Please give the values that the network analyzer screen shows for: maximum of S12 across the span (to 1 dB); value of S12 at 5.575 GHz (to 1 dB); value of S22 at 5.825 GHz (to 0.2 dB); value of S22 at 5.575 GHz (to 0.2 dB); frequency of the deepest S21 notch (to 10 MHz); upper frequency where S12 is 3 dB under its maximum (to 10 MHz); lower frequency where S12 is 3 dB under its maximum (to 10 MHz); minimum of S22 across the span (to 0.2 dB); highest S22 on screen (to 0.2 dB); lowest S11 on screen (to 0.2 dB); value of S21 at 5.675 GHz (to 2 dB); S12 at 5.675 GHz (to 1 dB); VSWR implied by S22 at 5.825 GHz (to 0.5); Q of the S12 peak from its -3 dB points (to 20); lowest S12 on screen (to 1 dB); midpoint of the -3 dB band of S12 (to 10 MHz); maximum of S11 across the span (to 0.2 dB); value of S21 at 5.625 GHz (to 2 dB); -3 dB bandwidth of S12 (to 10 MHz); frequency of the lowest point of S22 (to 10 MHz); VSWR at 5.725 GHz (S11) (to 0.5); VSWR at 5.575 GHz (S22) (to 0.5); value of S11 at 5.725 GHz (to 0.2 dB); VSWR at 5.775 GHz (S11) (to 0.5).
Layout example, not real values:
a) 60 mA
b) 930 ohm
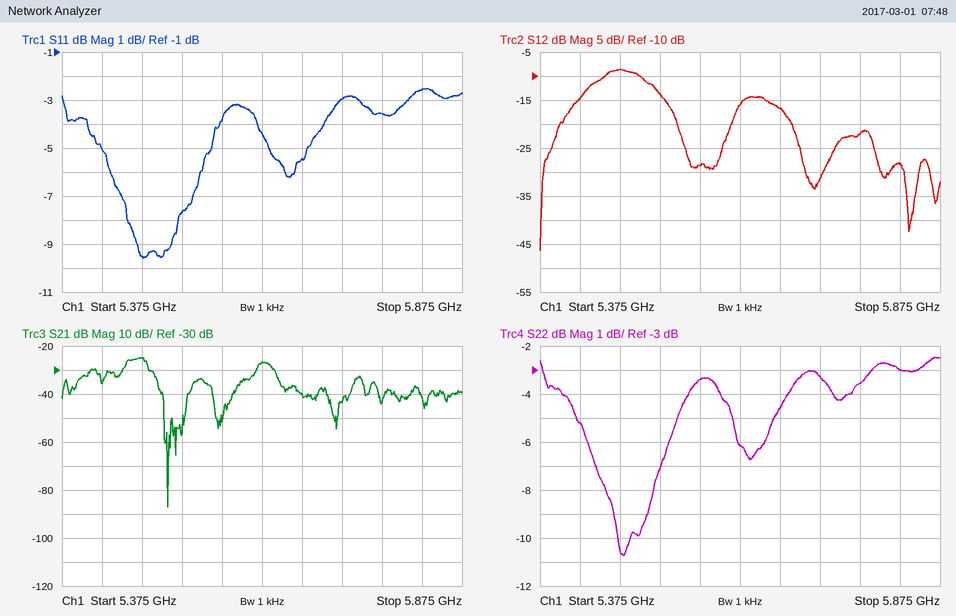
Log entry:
a) -9 dB
b) -29 dB
c) -3.0 dB
d) -3.4 dB
e) 5.51 GHz
f) 5.51 GHz
g) 5.44 GHz
h) -10.8 dB
i) -2.4 dB
j) -9.6 dB
k) -40 dB
l) -17 dB
m) 6.0
n) 80
o) -46 dB
p) 5.48 GHz
q) -2.6 dB
r) -26 dB
s) 70 MHz
t) 5.48 GHz
u) 6.0
v) 5.0
w) -3.0 dB
x) 5.0
